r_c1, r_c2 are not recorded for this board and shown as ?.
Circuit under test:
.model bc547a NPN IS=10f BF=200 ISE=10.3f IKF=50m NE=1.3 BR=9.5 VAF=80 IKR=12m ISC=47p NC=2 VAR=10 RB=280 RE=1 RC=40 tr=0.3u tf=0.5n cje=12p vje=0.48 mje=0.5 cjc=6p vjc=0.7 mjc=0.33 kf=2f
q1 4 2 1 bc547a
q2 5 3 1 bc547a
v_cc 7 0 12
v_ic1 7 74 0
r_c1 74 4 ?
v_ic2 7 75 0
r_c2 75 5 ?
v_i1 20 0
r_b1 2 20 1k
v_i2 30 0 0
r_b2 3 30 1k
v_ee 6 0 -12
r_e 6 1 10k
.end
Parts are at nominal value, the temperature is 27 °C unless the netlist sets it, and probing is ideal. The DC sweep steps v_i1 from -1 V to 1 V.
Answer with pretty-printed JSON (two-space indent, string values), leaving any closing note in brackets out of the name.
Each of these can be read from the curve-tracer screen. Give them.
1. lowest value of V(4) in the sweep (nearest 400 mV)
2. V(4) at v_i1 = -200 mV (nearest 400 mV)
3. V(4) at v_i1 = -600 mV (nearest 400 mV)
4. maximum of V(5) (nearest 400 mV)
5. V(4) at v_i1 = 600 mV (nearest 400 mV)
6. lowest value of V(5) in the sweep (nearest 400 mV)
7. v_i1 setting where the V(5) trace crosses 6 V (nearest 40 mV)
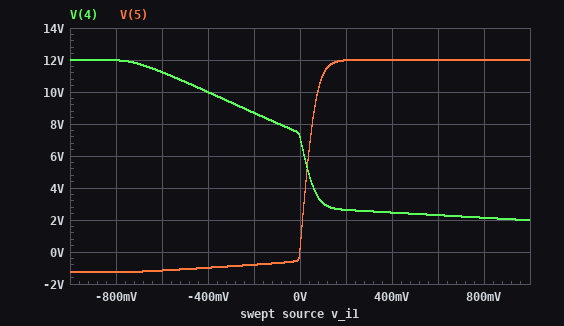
{
  "lowest value of V(4) in the sweep": "2.0 V",
  "V(4) at v_i1 = -200 mV": "8.8 V",
  "V(4) at v_i1 = -600 mV": "11.2 V",
  "maximum of V(5)": "12.0 V",
  "V(4) at v_i1 = 600 mV": "2.4 V",
  "lowest value of V(5) in the sweep": "-1.2 V",
  "v_i1 setting where the V(5) trace crosses 6 V": "40 mV"
}
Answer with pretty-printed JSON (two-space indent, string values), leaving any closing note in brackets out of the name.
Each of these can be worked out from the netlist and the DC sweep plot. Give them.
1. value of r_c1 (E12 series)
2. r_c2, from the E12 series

{
  "value of r_c1": "8.2 kΩ",
  "r_c2, from the E12 series": "22 kΩ"
}
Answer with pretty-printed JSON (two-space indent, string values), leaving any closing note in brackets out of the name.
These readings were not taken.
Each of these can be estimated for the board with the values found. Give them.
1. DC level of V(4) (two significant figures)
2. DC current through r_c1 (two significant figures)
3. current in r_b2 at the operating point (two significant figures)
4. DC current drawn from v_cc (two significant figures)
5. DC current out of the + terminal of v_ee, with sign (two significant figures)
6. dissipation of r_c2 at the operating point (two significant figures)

{
  "DC level of V(4)": "7.2 V",
  "DC current through r_c1": "590 µA",
  "current in r_b2 at the operating point": "4.9 µA",
  "DC current drawn from v_cc": "1.1 mA",
  "DC current out of the + terminal of v_ee, with sign": "-1.1 mA",
  "dissipation of r_c2 at the operating point": "6.4 mW"
}
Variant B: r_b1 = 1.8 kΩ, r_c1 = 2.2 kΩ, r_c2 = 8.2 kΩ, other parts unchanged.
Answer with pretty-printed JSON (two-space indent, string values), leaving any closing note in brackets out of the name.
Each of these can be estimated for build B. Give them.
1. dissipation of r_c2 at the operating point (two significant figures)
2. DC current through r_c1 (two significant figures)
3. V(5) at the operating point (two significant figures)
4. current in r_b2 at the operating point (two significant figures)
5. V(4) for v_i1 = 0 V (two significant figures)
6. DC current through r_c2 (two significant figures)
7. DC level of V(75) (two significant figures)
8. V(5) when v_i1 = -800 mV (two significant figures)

{
  "dissipation of r_c2 at the operating point": "2.8 mW",
  "DC current through r_c1": "540 µA",
  "V(5) at the operating point": "7.2 V",
  "current in r_b2 at the operating point": "4.8 µA",
  "V(4) for v_i1 = 0 V": "11 V",
  "DC current through r_c2": "580 µA",
  "DC level of V(75)": "12 V",
  "V(5) when v_i1 = -800 mV": "2.8 V"
}
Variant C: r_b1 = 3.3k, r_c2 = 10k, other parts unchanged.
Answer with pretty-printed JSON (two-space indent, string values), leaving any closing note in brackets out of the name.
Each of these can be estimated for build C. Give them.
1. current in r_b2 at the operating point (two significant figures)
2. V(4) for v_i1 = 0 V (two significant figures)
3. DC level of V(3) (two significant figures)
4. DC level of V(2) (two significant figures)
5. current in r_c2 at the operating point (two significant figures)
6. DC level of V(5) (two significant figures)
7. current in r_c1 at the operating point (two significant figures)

{
  "current in r_b2 at the operating point": "5.3 µA",
  "V(4) for v_i1 = 0 V": "8.0 V",
  "DC level of V(3)": "-5.3 mV",
  "DC level of V(2)": "-13 mV",
  "current in r_c2 at the operating point": "640 µA",
  "DC level of V(5)": "5.6 V",
  "current in r_c1 at the operating point": "490 µA"
}
